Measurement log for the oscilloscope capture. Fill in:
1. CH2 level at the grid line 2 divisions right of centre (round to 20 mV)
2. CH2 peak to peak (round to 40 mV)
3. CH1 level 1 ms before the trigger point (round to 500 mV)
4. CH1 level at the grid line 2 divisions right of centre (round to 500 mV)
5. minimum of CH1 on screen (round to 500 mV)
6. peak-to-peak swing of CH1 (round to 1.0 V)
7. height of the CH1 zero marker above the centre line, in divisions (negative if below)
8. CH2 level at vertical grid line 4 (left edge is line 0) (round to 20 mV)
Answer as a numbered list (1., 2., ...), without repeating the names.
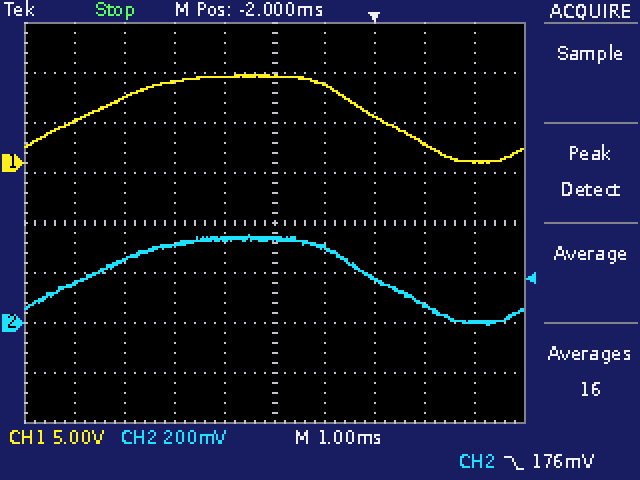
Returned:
1. 180 mV
2. 360 mV
3. 8.0 V
4. 4.5 V
5. 0.0 V
6. 9.0 V
7. +1.2 div
8. 340 mV
